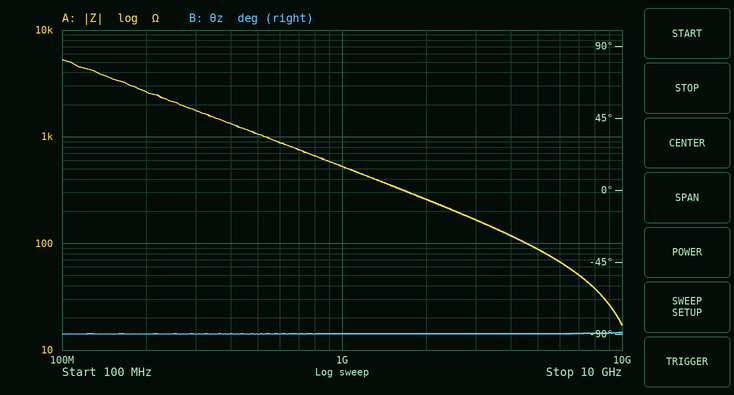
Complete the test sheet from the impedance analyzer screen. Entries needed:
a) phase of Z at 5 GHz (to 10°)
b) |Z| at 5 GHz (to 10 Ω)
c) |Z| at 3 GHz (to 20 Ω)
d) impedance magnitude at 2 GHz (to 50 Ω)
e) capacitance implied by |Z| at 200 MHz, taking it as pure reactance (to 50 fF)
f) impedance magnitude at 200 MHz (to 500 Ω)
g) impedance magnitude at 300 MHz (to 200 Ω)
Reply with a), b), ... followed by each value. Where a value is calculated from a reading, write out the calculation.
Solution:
a) -90°
b) 90 Ω
c) 160 Ω
d) 250 Ω
e) C = 1/(2π × 200 MHz × 2.5 kΩ) ≈ 318 fF, so 300 fF to the nearest 50 fF
f) 2.5 kΩ
g) 1.8 kΩ
